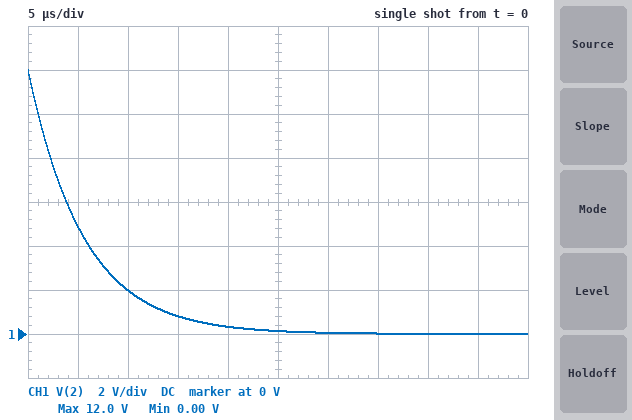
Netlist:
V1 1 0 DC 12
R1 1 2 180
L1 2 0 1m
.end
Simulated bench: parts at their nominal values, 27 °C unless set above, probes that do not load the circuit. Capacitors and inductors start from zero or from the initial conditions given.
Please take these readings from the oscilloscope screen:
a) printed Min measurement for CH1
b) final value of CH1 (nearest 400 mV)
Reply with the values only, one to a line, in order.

0.00 V
0 V
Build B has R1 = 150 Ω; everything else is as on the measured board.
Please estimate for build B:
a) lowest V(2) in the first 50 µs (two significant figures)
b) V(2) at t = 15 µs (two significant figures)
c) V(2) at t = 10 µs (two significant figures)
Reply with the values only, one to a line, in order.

6.6 mV
1.3 V
2.7 V
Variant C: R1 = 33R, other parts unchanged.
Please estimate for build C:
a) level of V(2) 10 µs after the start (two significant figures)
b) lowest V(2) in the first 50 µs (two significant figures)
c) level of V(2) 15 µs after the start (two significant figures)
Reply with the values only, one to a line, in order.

8.6 V
2.3 V
7.3 V
